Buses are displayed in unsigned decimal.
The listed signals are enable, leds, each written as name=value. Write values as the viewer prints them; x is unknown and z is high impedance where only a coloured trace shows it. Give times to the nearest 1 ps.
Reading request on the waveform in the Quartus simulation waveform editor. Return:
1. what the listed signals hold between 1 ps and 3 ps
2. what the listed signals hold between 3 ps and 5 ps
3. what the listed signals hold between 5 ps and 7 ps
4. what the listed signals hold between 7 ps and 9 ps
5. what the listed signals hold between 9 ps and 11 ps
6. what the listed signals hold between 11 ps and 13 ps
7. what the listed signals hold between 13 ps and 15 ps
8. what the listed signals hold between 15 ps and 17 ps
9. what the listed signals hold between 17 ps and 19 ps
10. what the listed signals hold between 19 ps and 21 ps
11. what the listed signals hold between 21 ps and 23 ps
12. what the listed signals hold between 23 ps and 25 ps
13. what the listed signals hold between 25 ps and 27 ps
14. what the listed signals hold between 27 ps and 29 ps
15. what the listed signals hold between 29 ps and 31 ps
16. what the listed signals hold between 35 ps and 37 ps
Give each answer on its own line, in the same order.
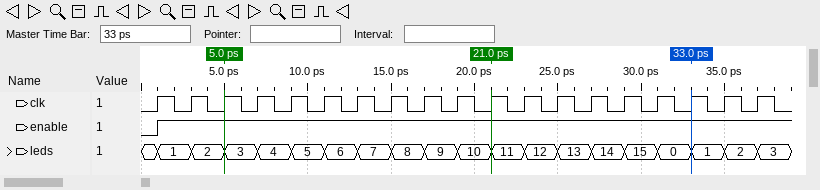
enable=1, leds=1
enable=1, leds=2
enable=1, leds=3
enable=1, leds=4
enable=1, leds=5
enable=1, leds=6
enable=1, leds=7
enable=1, leds=8
enable=1, leds=9
enable=1, leds=10
enable=1, leds=11
enable=1, leds=12
enable=1, leds=13
enable=1, leds=14
enable=1, leds=15
enable=1, leds=2
